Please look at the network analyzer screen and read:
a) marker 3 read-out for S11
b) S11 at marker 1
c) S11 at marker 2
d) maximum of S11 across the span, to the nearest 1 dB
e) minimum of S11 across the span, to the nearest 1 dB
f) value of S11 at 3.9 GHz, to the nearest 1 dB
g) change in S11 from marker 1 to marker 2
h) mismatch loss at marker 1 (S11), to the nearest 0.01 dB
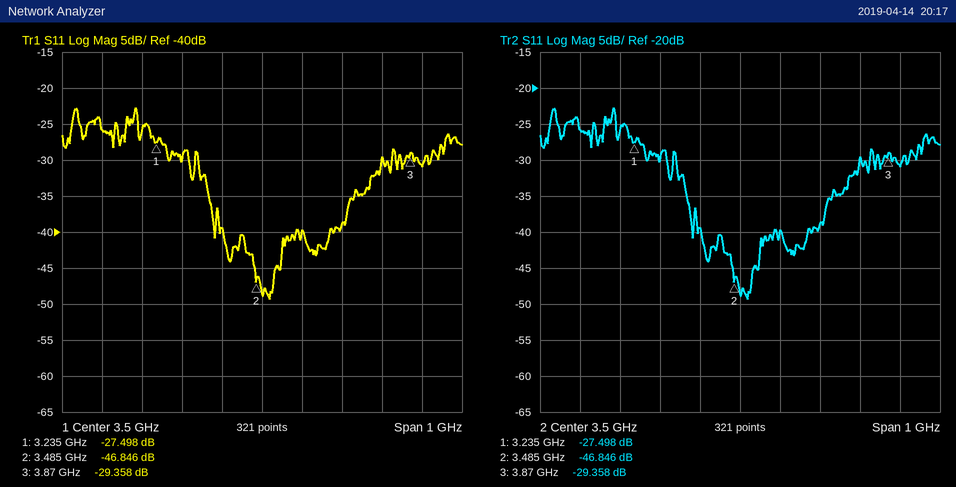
-29.358 dB
-27.498 dB
-46.846 dB
-23 dB
-49 dB
-31 dB
-19.348 dB
0.01 dB
